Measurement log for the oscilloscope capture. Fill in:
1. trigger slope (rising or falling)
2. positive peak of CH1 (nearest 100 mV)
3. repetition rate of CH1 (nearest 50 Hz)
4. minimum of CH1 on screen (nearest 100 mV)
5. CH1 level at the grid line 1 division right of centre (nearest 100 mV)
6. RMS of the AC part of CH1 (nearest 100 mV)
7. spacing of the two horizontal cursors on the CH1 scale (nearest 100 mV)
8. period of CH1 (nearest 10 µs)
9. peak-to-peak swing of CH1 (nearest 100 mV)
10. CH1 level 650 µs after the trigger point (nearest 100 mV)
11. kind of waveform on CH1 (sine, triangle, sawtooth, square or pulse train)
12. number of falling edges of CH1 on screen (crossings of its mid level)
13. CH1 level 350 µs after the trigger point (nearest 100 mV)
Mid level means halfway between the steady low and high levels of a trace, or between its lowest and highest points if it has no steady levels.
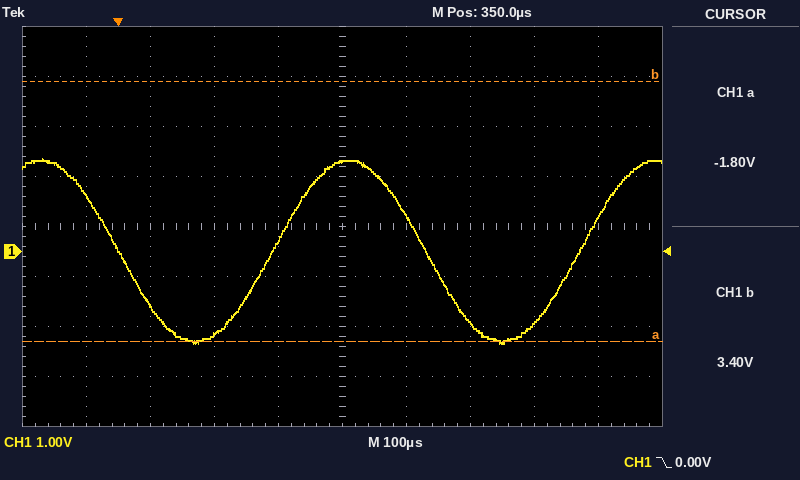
falling
1.9 V
2.10 kHz
-1.8 V
700 mV
1.3 V
5.2 V
480 µs
3.7 V
-1.4 V
sine
2
1.8 V
